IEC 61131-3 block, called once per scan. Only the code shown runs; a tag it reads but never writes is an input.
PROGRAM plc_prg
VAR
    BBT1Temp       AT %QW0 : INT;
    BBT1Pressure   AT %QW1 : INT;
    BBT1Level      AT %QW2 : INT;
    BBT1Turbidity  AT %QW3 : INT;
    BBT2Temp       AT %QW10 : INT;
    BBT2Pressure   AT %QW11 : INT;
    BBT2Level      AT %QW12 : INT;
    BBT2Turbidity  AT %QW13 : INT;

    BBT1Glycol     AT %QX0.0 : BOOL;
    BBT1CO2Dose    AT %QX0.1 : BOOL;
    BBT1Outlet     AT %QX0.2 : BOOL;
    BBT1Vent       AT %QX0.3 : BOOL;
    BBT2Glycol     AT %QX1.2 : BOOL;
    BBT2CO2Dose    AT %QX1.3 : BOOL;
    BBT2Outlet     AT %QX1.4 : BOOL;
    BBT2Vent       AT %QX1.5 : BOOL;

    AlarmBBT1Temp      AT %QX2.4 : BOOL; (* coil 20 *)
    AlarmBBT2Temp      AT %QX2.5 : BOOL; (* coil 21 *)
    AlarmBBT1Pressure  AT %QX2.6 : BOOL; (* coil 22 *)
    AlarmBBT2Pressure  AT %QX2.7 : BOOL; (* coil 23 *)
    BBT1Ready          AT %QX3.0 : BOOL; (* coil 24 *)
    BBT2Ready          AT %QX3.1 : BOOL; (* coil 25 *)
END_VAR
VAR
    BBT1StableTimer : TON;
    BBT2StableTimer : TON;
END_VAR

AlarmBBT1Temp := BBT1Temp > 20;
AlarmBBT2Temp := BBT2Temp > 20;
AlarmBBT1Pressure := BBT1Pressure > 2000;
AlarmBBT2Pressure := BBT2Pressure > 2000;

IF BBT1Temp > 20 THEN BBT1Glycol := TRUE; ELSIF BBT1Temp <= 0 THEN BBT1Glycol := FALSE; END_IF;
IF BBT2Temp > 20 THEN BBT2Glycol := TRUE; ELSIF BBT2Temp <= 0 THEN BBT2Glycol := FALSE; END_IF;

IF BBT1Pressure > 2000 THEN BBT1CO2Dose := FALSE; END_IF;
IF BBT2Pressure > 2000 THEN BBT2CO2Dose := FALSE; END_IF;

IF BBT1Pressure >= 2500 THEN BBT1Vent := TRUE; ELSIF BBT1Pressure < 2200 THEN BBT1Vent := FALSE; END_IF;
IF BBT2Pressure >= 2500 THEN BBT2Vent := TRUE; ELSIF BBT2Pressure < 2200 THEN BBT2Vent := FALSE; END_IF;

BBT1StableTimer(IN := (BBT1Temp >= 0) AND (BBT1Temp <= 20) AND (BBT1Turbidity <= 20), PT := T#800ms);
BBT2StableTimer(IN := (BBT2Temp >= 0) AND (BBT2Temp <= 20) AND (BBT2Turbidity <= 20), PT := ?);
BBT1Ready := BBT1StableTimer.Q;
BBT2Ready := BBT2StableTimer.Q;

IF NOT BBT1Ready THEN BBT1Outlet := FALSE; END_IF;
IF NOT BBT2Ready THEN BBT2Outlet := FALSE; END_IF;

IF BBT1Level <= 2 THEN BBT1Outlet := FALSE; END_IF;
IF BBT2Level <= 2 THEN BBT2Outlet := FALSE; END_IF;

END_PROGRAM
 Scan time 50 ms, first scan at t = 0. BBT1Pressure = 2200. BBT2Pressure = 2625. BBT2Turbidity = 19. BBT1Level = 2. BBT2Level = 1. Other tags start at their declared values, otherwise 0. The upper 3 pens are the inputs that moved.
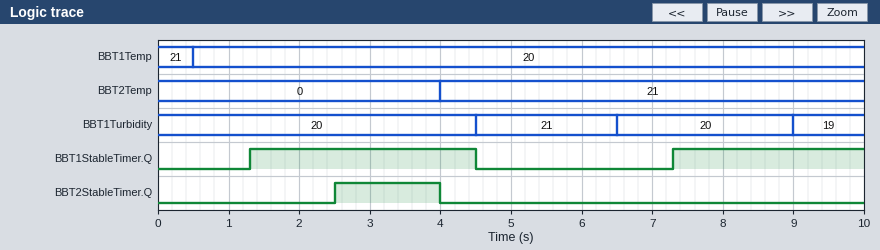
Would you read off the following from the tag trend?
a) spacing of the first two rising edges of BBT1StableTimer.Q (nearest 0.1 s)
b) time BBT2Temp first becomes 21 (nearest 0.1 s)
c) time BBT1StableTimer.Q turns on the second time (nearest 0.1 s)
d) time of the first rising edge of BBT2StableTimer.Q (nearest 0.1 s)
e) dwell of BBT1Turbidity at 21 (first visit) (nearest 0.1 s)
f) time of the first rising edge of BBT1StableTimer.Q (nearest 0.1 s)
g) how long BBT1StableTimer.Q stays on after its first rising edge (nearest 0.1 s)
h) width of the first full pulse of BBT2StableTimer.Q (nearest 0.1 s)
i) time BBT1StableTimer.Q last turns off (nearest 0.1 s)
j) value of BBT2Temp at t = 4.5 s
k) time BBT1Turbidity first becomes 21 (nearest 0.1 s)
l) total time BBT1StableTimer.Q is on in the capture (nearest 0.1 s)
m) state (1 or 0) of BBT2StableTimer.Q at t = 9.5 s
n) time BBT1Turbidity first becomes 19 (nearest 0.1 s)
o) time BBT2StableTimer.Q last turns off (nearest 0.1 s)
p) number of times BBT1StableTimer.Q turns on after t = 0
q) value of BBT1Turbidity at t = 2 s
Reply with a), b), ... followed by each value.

a) 6.0 s
b) 4.0 s
c) 7.3 s
d) 2.5 s
e) 2.0 s
f) 1.3 s
g) 3.2 s
h) 1.5 s
i) 4.5 s
j) 21
k) 4.5 s
l) 5.9 s
m) 0
n) 9.0 s
o) 4.0 s
p) 2
q) 20
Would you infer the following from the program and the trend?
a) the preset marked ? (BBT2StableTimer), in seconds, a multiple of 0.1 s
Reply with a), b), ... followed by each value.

a) 2.5 s
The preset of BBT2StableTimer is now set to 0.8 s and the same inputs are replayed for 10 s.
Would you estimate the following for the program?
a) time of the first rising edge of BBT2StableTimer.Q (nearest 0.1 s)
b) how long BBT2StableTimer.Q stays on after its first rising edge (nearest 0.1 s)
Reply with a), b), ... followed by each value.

a) 0.8 s
b) 3.2 s
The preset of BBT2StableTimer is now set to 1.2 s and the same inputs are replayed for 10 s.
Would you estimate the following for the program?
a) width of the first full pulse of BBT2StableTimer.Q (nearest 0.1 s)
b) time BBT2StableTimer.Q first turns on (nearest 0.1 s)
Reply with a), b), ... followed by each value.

a) 2.8 s
b) 1.2 s
